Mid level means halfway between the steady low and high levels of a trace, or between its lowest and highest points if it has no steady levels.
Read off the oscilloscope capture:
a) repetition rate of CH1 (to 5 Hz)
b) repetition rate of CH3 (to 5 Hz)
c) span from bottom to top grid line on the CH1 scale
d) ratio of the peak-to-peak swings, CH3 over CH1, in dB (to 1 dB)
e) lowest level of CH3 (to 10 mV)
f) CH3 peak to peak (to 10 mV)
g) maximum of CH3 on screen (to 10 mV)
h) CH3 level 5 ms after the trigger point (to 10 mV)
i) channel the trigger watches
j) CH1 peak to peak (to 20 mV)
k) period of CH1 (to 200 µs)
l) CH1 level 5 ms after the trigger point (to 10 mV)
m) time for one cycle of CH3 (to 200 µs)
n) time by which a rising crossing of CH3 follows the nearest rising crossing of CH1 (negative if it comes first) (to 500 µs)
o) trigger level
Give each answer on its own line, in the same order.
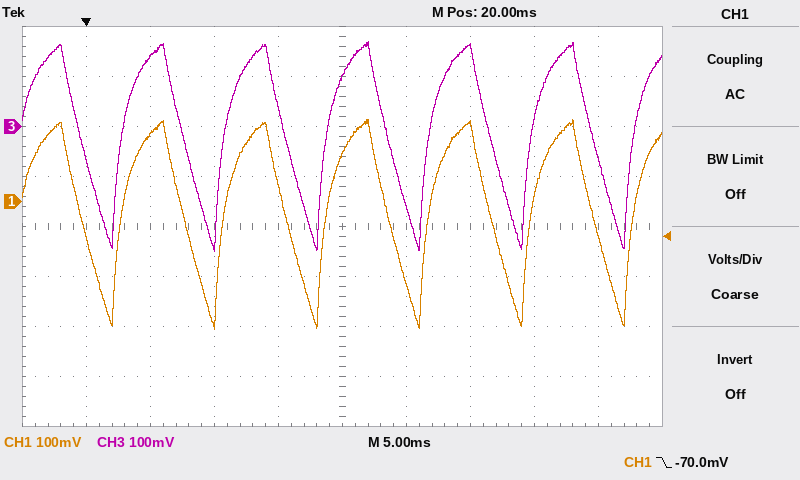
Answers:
125 Hz
125 Hz
800 mV
0 dB
-250 mV
420 mV
170 mV
140 mV
CH1
420 mV
8.0 ms
130 mV
8.0 ms
0.0 ms
-70.0 mV
